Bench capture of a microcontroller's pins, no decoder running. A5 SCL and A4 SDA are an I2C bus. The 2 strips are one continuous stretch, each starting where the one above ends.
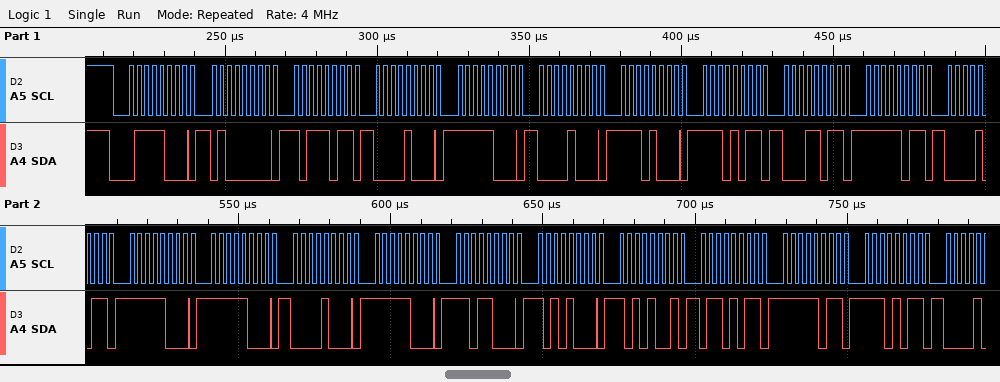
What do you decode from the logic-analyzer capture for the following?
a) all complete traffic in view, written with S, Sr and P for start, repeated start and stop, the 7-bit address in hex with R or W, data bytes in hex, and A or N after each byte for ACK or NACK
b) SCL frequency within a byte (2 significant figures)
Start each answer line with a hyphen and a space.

- S 3CW A 40 A BB A 08 A F8 A 08 A E8 A EB A 1B A FB A 0B A F8 A F8 A 08 A F8 A D8 A A8 A A9 A 6B A FB A EB A
- 400 kHz
